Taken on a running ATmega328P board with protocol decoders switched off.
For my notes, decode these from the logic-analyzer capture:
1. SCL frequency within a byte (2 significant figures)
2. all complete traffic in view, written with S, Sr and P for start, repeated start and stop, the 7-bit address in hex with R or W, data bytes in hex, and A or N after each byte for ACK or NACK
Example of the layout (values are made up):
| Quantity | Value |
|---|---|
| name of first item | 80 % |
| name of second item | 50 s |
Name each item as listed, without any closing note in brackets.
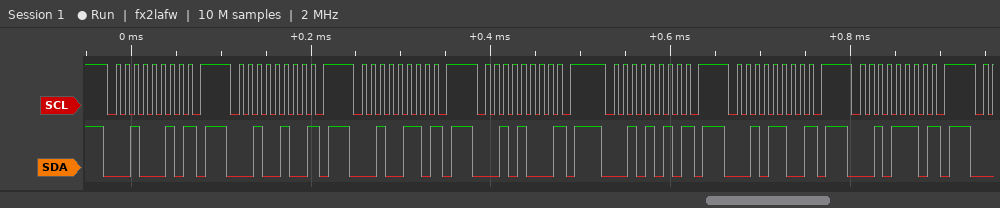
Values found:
| Quantity | Value |
|---|---|
| SCL frequency within a byte | 100 kHz |
| all complete traffic in view, written with S, Sr and P for start, repeated start and stop, the 7-bit address in hex with R or W, data bytes in hex, and A or N after each byte for ACK or NACK | S 11W N P S 12W N P S 13W N P S 14W N P S 15W N P S 16W N P S 17W N P |
